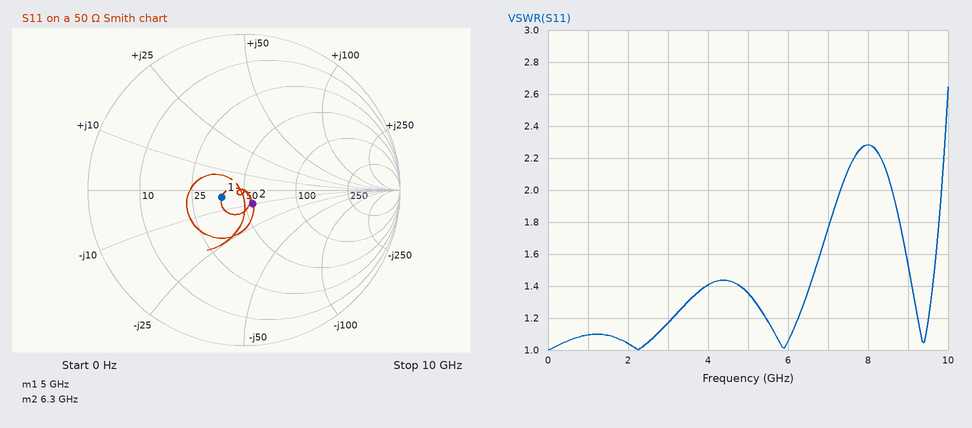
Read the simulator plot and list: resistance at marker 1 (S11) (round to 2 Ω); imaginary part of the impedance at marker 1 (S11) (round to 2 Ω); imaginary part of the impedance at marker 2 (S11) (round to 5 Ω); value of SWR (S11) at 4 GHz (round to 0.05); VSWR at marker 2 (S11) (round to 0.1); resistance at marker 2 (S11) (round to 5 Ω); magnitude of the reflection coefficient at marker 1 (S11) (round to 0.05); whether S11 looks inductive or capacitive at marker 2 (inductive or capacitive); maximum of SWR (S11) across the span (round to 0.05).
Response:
38 Ω
-4 Ω
-10 Ω
1.40
1.2
55 Ω
0.15
capacitive
2.65
